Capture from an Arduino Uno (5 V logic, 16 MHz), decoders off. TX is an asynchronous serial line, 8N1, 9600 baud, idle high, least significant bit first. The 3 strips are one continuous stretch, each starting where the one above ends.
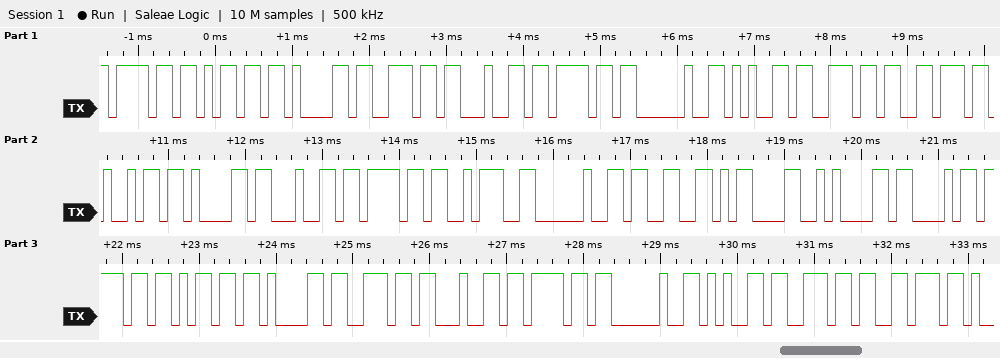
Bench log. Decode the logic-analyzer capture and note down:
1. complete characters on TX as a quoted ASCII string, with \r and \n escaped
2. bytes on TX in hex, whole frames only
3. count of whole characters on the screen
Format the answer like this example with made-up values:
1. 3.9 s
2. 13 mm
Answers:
1. "omando enviado: 3\r\nComando env"
2. 6F 6D 61 6E 64 6F 20 65 6E 76 69 61 64 6F 3A 20 33 0D 0A 43 6F 6D 61 6E 64 6F 20 65 6E 76
3. 30
